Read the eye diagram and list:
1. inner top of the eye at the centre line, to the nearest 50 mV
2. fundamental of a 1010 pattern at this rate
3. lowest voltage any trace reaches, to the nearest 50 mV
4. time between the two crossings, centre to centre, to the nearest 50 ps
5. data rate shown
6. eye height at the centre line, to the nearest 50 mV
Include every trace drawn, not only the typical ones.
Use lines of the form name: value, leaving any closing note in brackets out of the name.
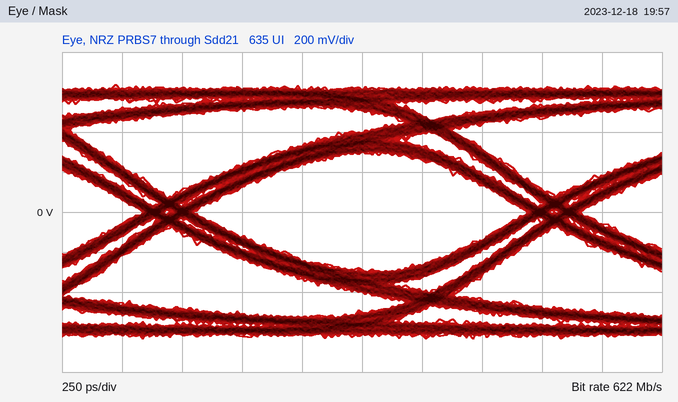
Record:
inner top of the eye at the centre line, to the nearest 50 mV: 300 mV
fundamental of a 1010 pattern at this rate: 311 MHz
lowest voltage any trace reaches, to the nearest 50 mV: -650 mV
time between the two crossings, centre to centre, to the nearest 50 ps: 1.60 ns
data rate shown: 622 Mb/s
eye height at the centre line, to the nearest 50 mV: 600 mV
